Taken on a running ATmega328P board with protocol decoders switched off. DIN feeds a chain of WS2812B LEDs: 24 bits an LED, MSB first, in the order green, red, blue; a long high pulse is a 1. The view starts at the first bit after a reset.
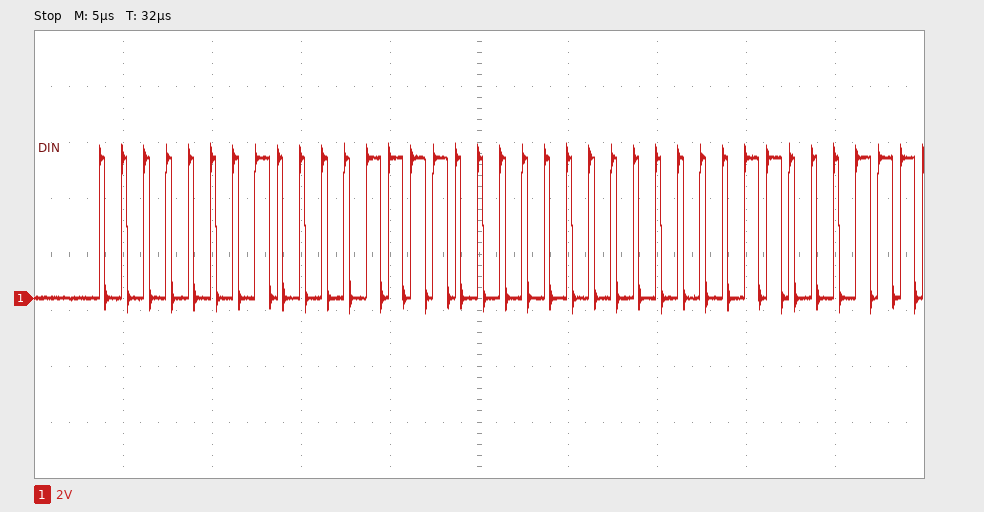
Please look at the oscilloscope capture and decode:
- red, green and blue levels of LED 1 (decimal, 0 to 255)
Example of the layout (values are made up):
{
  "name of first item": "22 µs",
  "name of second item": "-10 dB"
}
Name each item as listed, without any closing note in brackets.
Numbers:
{
  "red, green and blue levels of LED 1": "15, 1, 0"
}
